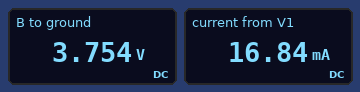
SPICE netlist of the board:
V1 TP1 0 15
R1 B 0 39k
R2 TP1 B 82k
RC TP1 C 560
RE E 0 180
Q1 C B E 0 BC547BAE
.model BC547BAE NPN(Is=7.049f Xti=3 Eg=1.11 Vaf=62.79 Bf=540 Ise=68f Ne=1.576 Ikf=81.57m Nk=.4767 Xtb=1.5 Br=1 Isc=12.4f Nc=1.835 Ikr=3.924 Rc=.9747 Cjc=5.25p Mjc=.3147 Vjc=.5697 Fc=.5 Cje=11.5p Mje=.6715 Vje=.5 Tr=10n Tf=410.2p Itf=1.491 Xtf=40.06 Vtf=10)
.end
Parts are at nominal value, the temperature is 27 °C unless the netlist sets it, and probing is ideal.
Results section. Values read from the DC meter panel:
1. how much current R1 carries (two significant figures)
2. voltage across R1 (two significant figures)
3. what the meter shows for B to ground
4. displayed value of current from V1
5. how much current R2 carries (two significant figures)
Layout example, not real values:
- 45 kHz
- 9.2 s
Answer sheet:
- 96 µA
- 3.8 V
- 3.754 V
- 16.84 mA
- 140 µA
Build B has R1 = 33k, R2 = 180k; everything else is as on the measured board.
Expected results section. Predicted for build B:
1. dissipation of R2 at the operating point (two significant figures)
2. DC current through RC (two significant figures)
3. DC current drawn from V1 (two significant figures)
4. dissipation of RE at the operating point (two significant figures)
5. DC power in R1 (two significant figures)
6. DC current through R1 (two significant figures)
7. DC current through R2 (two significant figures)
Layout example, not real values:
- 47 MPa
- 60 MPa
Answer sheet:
- 950 µW
- 6.7 mA
- 6.8 mA
- 8.2 mW
- 110 µW
- 58 µA
- 73 µA
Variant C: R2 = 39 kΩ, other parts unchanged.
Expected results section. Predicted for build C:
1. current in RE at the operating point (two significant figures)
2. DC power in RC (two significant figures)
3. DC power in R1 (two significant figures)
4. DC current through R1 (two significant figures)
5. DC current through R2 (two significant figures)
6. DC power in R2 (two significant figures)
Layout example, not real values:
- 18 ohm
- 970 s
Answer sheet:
- 20 mA
- 220 mW
- 490 µW
- 110 µA
- 270 µA
- 2.9 mW
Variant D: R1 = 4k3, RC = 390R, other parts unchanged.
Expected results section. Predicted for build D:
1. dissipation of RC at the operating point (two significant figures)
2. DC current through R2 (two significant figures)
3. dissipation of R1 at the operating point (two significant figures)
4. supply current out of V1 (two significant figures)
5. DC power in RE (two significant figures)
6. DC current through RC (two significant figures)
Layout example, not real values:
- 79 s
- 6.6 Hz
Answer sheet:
- 120 µW
- 170 µA
- 130 µW
- 720 µA
- 54 µW
- 550 µA
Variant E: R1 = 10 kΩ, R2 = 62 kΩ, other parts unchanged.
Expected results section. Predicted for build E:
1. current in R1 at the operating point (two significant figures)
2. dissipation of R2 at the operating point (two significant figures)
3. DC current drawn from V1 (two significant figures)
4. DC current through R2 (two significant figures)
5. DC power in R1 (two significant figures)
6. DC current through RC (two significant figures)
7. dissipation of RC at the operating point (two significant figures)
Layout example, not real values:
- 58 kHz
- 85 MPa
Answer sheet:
- 200 µA
- 2.7 mW
- 7.1 mA
- 210 µA
- 380 µW
- 6.9 mA
- 27 mW
